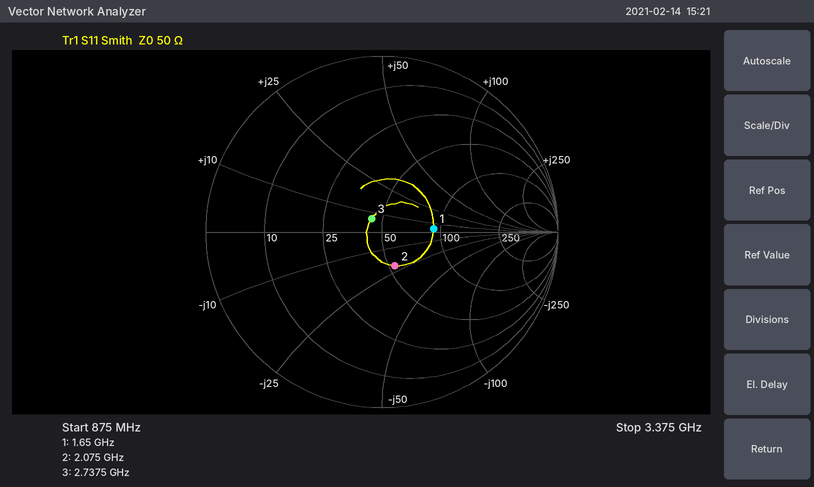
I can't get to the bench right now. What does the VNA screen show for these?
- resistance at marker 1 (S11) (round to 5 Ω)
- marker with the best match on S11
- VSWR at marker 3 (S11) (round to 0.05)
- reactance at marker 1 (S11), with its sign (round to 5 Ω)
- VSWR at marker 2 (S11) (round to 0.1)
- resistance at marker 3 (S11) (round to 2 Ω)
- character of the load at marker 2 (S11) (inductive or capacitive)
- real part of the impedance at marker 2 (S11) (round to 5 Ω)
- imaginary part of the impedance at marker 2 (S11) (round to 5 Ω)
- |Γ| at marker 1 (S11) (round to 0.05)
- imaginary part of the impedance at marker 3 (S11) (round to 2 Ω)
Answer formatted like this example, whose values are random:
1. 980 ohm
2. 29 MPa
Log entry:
1. 90 Ω
2. marker 3
3. 1.20
4. +5 Ω
5. 1.5
6. 44 Ω
7. capacitive
8. 55 Ω
9. -20 Ω
10. 0.30
11. +6 Ω
